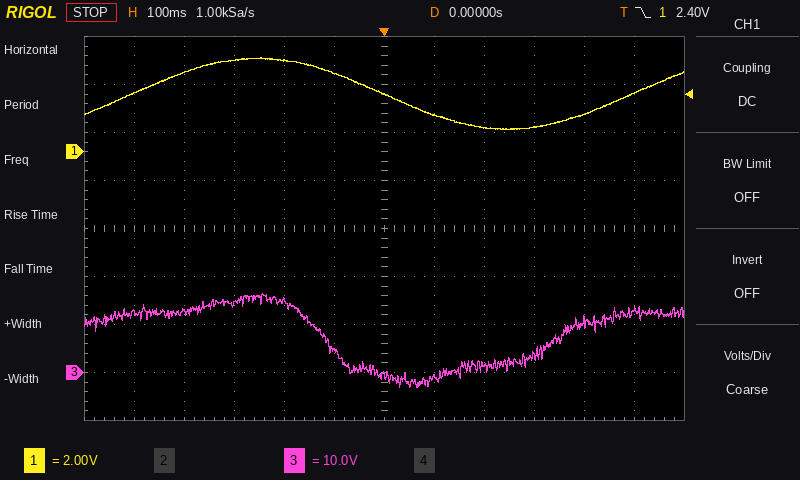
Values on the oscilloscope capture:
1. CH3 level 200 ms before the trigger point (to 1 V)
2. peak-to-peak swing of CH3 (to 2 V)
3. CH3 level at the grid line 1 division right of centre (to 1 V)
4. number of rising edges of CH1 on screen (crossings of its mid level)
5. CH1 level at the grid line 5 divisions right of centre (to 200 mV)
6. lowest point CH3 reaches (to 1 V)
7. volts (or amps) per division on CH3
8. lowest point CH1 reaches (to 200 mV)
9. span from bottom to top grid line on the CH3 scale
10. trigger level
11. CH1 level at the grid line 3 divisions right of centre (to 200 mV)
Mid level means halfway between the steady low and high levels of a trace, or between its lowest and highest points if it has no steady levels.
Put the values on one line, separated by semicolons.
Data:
15 V; 20 V; -1 V; 2; 2.4 V; -3 V; 10 V; 1.0 V; 80 V; 2.40 V; 1.0 V
